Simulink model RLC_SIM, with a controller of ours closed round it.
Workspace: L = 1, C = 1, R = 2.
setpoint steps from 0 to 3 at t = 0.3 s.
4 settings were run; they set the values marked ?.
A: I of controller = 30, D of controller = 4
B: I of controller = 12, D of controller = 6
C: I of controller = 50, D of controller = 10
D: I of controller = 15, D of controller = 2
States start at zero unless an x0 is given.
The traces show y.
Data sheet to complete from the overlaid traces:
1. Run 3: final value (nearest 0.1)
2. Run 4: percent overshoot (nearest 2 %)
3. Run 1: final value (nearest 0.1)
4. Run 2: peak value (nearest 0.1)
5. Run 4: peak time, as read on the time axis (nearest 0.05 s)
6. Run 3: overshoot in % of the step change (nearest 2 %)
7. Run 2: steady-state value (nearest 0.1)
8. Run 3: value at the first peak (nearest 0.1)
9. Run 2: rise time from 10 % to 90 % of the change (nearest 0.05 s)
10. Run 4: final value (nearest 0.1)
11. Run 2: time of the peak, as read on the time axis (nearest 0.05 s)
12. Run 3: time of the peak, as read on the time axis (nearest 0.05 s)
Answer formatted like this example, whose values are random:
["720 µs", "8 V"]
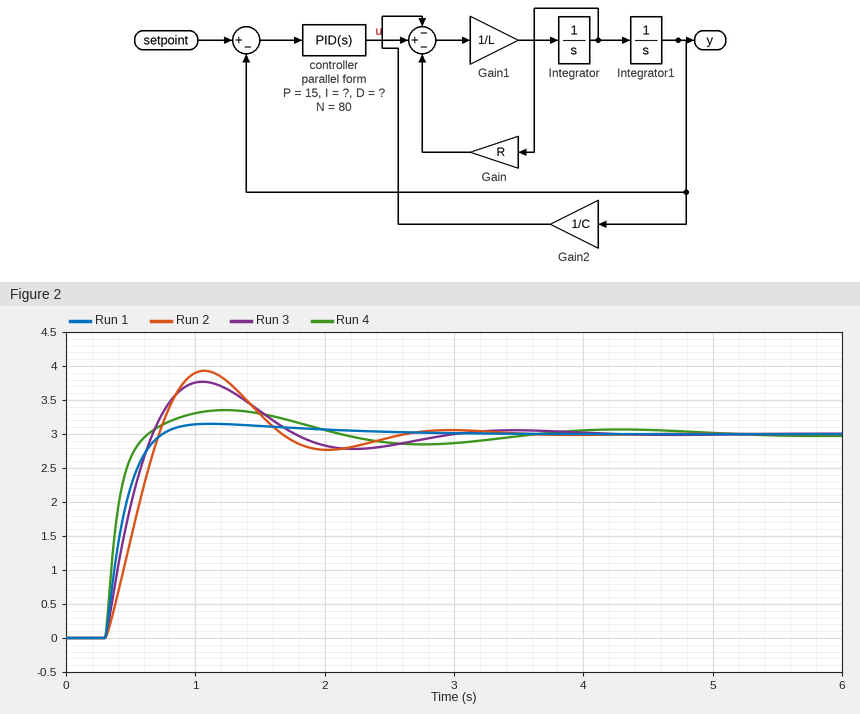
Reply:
["3.0", "12 %", "3.0", "3.9", "1.25 s", "26 %", "3.0", "3.8", "0.30 s", "3.0", "1.05 s", "1.05 s"]
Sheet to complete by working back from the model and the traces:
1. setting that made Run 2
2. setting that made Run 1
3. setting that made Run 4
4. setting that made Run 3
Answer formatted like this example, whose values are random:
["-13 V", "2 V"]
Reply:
["D", "B", "C", "A"]
